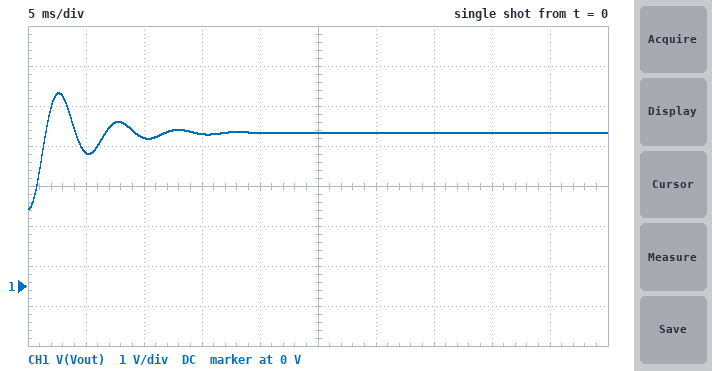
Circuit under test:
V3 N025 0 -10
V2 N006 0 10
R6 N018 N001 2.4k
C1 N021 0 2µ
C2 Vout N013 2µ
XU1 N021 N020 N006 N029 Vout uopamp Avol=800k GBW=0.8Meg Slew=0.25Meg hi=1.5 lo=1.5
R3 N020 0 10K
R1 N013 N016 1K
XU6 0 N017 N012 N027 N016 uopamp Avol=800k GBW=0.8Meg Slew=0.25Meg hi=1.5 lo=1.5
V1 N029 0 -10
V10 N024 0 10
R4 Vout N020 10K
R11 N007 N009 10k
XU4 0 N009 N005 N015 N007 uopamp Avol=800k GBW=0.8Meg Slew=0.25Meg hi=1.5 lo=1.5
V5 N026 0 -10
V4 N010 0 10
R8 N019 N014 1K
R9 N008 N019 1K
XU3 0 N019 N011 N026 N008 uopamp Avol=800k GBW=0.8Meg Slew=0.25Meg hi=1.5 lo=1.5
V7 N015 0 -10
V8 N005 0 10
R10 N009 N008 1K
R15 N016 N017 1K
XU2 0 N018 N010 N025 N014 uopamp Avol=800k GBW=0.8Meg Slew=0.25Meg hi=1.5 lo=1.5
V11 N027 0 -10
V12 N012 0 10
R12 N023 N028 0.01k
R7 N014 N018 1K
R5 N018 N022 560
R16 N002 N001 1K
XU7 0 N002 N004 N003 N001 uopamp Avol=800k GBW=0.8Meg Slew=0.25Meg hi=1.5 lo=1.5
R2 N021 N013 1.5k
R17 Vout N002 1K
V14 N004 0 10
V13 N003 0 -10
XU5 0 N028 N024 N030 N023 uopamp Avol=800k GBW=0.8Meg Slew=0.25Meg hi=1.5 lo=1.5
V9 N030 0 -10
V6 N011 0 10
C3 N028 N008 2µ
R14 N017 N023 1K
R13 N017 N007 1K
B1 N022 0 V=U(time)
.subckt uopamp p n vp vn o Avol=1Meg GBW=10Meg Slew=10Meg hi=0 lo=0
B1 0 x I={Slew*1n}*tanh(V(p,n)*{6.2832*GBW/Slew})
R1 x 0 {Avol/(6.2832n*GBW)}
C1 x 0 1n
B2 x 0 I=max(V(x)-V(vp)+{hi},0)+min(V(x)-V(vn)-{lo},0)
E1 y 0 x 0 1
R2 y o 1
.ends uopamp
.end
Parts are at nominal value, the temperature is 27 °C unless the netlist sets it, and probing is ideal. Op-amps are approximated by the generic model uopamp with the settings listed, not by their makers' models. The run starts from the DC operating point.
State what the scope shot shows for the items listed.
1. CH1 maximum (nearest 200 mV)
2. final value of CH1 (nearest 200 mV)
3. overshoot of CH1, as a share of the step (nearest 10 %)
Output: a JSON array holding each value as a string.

["4.8 V", "3.8 V", "50 %"]
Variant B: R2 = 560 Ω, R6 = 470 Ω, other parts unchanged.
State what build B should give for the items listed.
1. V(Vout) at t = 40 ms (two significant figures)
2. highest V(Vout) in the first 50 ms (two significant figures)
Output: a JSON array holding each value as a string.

["820 mV", "1.2 V"]
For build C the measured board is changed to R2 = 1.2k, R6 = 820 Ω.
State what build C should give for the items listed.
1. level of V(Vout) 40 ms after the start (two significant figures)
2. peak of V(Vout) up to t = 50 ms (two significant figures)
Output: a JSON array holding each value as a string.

["1.4 V", "1.9 V"]
